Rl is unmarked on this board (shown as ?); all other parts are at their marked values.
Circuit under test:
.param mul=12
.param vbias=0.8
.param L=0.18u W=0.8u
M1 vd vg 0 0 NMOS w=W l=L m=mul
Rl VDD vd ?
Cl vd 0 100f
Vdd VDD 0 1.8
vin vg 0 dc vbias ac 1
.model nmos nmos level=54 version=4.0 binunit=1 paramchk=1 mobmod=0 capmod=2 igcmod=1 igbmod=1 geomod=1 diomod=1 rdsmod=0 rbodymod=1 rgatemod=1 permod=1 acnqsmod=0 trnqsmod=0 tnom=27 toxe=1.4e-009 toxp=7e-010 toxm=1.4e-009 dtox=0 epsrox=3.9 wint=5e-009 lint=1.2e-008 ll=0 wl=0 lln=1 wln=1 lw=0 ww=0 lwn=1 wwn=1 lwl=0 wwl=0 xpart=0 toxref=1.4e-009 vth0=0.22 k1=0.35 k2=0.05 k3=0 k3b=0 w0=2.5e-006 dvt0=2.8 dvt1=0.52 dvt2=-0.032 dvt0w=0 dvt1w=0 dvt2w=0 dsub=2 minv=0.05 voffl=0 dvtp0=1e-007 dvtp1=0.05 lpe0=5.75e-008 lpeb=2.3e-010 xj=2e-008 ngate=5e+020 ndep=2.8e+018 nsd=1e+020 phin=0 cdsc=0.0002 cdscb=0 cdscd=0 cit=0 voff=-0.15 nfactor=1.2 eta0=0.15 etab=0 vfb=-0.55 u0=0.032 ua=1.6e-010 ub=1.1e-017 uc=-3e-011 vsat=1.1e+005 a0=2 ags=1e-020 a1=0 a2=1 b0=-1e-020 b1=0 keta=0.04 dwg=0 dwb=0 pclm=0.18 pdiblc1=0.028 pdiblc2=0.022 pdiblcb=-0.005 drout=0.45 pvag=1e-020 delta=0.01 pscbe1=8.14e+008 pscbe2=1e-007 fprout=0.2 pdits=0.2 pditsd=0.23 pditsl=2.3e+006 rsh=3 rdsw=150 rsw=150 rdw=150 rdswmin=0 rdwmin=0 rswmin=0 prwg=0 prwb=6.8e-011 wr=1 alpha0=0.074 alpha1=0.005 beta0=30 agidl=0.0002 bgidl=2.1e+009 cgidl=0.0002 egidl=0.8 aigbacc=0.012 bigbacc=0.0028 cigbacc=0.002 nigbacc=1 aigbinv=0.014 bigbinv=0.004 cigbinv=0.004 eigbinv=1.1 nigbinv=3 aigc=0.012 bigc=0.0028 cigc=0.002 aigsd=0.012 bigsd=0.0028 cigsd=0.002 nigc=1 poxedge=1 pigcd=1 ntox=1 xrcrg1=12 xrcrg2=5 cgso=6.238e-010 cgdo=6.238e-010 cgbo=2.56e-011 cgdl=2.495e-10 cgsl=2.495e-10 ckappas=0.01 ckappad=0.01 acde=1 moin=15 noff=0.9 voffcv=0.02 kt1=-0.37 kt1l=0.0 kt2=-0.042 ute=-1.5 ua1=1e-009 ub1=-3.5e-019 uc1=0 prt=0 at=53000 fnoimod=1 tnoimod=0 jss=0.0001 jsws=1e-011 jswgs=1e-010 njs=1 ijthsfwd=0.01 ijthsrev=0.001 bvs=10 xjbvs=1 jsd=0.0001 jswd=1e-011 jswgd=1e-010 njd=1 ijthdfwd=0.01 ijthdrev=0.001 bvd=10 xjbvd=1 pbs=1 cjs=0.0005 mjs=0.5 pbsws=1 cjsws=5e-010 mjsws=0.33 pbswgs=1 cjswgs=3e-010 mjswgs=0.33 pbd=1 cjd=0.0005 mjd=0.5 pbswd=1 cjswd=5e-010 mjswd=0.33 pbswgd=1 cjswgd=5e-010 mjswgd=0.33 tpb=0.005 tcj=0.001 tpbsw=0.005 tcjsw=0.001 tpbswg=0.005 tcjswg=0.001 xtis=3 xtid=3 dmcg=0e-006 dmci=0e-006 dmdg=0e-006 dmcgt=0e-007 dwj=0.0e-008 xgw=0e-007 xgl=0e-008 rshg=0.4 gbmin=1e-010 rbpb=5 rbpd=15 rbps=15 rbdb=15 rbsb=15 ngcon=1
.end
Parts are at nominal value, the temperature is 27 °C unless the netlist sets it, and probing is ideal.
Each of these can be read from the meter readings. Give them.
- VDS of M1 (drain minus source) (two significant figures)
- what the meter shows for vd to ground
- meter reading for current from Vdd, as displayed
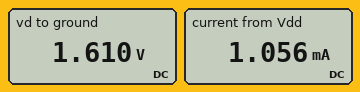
1.6 V
1.610 V
1.056 mA
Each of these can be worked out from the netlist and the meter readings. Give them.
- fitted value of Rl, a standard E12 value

180 Ω
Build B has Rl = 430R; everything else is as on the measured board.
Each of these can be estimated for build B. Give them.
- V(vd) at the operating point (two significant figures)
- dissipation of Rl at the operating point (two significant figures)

1.4 V
450 µW
